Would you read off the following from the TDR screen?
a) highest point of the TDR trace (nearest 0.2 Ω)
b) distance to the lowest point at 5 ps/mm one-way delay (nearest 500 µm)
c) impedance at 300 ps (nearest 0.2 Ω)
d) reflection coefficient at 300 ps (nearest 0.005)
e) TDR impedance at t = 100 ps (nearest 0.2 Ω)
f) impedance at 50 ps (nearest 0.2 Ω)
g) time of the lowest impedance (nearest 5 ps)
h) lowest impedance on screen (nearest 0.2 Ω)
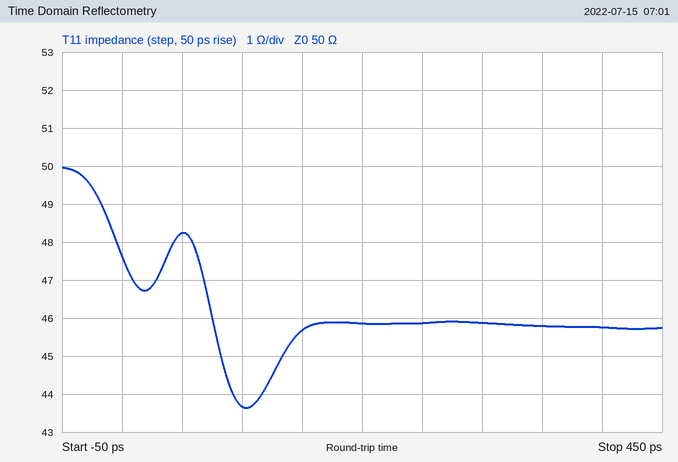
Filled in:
50.0 Ω
10.5 mm
45.8 Ω
-0.045
43.6 Ω
48.2 Ω
105 ps
43.6 Ω
